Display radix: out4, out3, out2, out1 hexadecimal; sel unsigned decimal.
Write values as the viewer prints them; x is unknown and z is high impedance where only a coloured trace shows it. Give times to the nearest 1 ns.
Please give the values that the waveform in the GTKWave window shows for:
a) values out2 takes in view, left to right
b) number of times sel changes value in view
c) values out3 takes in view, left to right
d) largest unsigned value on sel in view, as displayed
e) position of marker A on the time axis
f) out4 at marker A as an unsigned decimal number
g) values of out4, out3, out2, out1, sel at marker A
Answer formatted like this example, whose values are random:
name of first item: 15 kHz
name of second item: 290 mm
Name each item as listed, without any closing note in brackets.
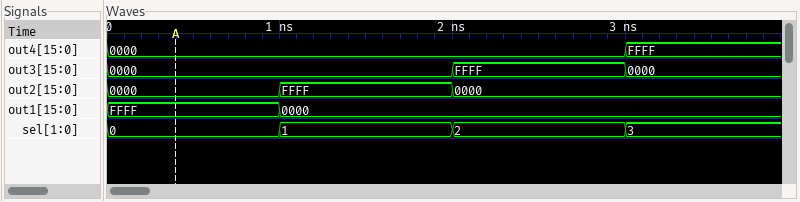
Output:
values out2 takes in view, left to right: 0000, FFFF, 0000
number of times sel changes value in view: 3
values out3 takes in view, left to right: 0000, FFFF, 0000
largest unsigned value on sel in view, as displayed: 3
position of marker A on the time axis: 0 ns
out4 at marker A as an unsigned decimal number: 0
values of out4, out3, out2, out1, sel at marker A: out4=0000, out3=0000, out2=0000, out1=FFFF, sel=0
